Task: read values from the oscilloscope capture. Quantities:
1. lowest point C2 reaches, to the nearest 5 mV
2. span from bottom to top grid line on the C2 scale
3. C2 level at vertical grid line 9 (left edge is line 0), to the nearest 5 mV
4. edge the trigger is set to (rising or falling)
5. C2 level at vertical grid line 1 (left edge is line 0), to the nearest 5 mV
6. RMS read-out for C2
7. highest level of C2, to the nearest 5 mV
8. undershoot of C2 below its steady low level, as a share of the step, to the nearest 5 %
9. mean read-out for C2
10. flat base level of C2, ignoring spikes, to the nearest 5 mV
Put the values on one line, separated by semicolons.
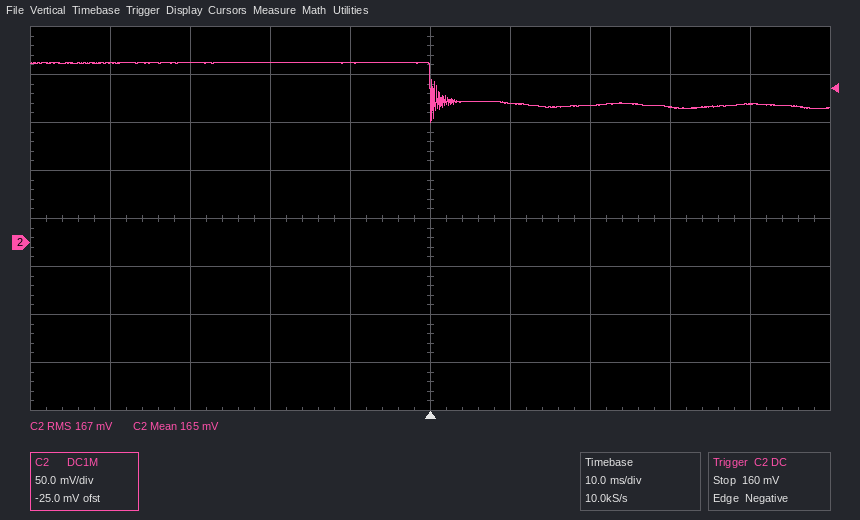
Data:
125 mV; 400 mV; 145 mV; falling; 185 mV; 167 mV; 190 mV; 40 %; 165 mV; 145 mV
